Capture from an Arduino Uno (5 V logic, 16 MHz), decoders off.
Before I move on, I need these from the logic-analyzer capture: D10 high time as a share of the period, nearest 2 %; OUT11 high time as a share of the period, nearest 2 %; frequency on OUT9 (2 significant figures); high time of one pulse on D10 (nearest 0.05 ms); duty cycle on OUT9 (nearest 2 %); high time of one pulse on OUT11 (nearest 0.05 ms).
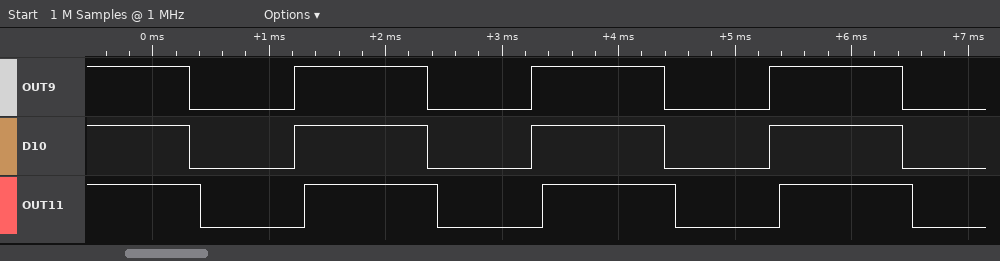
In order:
56 %
56 %
490 Hz
1.15 ms
56 %
1.15 ms
